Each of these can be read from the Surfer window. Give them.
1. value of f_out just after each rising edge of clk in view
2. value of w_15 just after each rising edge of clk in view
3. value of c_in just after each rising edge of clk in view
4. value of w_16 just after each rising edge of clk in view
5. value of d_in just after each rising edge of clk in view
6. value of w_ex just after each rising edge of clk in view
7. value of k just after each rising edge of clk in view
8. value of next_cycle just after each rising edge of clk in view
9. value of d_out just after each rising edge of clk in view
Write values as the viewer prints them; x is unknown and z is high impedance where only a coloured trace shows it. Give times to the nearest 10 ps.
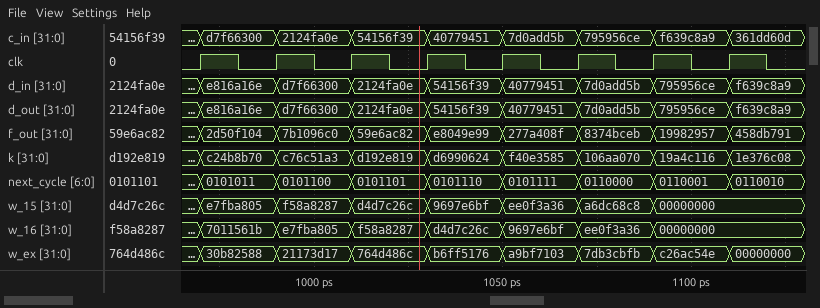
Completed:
2d50f104, 7b1096c0, 59e6ac82, e8049e99, 277a408f, 8374bceb, 19982957, 458db791
e7fba805, f58a8287, d4d7c26c, 9697e6bf, ee0f3a36, a6dc68c8, 00000000, 00000000
d7f66300, 2124fa0e, 54156f39, 40779451, 7d0add5b, 795956ce, f639c8a9, 361dd60d
7011561b, e7fba805, f58a8287, d4d7c26c, 9697e6bf, ee0f3a36, 00000000, 00000000
e816a16e, d7f66300, 2124fa0e, 54156f39, 40779451, 7d0add5b, 795956ce, f639c8a9
30b82588, 21173d17, 764d486c, b6ff5176, a9bf7103, 7db3cbfb, c26ac54e, 00000000
c24b8b70, c76c51a3, d192e819, d6990624, f40e3585, 106aa070, 19a4c116, 1e376c08
0101011, 0101100, 0101101, 0101110, 0101111, 0110000, 0110001, 0110010
e816a16e, d7f66300, 2124fa0e, 54156f39, 40779451, 7d0add5b, 795956ce, f639c8a9
